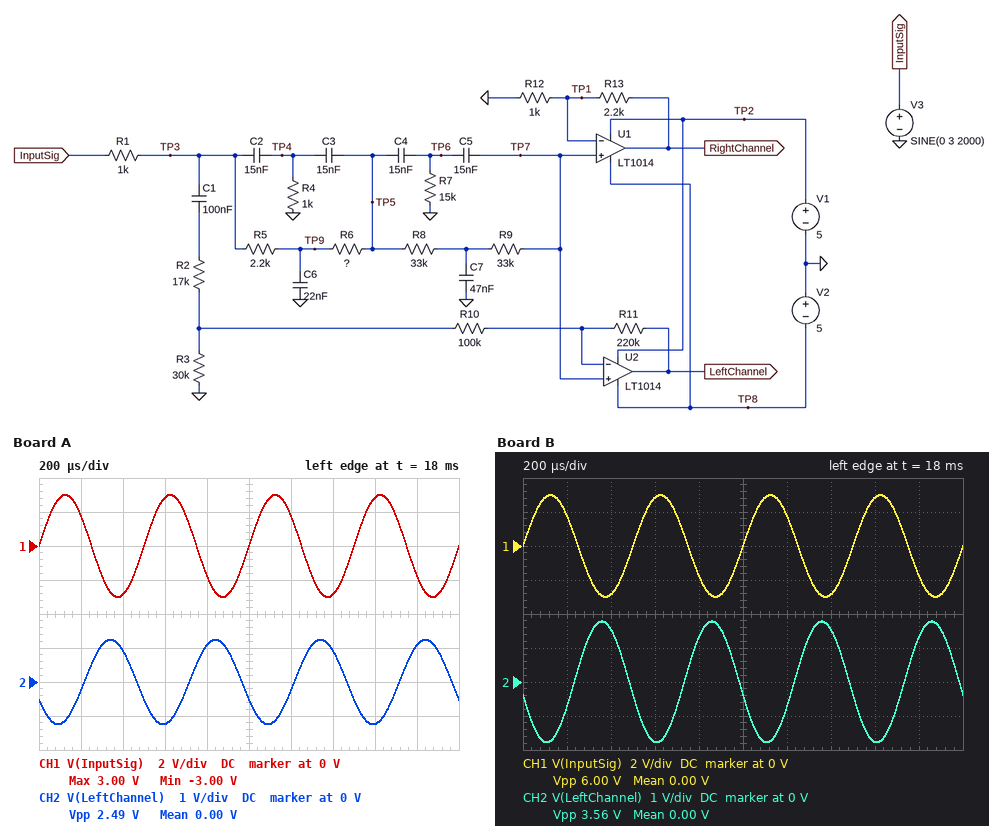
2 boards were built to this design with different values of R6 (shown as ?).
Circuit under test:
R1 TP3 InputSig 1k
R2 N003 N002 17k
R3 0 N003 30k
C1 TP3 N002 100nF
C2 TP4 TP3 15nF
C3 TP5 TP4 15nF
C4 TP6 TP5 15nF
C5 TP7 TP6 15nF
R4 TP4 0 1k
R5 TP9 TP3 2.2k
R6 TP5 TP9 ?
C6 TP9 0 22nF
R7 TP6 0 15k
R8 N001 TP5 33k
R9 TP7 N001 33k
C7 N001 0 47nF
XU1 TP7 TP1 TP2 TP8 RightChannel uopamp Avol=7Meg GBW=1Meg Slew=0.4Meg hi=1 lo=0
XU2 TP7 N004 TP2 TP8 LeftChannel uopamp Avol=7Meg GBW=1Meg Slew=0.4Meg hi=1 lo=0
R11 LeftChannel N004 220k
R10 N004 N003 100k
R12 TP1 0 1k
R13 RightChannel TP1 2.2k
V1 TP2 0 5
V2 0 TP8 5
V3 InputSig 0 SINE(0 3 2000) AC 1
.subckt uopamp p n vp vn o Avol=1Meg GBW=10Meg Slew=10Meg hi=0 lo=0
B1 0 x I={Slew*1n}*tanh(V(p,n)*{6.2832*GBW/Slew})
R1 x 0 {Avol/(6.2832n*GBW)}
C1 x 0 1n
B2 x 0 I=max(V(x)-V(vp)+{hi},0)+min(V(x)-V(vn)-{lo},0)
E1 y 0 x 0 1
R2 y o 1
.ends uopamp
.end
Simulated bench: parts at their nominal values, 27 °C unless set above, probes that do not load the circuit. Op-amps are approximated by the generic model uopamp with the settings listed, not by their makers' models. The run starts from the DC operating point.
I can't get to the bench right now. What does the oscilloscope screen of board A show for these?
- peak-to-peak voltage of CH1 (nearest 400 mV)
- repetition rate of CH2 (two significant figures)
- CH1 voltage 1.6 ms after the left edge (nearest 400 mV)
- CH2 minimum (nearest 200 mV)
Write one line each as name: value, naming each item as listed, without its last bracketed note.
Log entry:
peak-to-peak voltage of CH1: 6.0 V
repetition rate of CH2: 2.0 kHz
CH1 voltage 1.6 ms after the left edge: 2.8 V
CH2 minimum: -1.2 V
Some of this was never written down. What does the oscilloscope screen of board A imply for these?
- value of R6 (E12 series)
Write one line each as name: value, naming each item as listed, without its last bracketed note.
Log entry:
value of R6: 2.7 kΩ
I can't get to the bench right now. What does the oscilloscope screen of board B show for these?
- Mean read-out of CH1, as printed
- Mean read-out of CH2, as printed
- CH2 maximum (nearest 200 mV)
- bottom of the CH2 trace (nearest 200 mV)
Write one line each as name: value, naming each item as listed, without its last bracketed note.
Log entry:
Mean read-out of CH1, as printed: 0.00 V
Mean read-out of CH2, as printed: 0.00 V
CH2 maximum: 1.8 V
bottom of the CH2 trace: -1.8 V
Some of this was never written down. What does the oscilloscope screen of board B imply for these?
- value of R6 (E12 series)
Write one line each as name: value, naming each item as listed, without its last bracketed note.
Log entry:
value of R6: 4.7 kΩ
